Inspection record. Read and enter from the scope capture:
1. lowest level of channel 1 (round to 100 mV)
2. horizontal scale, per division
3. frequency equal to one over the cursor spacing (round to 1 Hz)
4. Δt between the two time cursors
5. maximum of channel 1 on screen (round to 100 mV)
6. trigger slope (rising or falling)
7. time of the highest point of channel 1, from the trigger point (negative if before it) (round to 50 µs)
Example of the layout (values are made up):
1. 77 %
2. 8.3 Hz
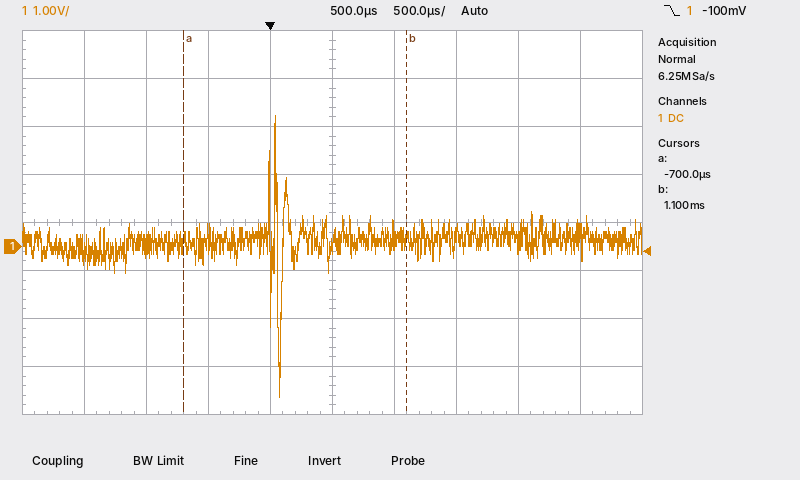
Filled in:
1. -3.1 V
2. 500 µs
3. 556 Hz
4. 1.80 ms
5. 2.7 V
6. falling
7. +50 µs
